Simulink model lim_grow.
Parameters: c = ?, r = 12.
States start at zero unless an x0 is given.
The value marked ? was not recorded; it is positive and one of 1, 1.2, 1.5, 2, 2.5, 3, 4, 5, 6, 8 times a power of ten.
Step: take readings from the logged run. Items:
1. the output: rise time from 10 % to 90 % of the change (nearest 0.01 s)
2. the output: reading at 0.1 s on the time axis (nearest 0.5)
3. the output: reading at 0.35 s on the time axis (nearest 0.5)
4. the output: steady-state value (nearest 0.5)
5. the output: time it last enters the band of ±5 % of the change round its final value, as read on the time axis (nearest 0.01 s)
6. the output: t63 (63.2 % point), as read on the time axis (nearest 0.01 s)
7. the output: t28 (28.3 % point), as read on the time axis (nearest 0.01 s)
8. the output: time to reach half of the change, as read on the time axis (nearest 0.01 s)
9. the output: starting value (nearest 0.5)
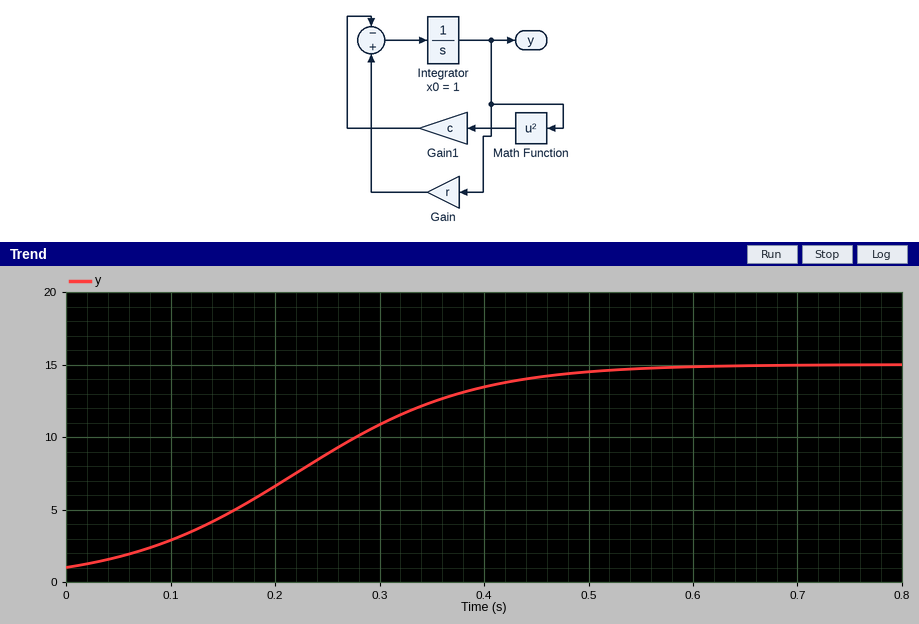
0.33 s
3.0
12.5
15.0
0.47 s
0.27 s
0.16 s
0.23 s
1.0
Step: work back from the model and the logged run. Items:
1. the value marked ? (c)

0.8
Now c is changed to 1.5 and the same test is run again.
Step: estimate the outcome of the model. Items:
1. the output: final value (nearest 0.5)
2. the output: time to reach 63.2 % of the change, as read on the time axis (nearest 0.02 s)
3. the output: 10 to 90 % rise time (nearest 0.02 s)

8.0
0.22 s
0.30 s
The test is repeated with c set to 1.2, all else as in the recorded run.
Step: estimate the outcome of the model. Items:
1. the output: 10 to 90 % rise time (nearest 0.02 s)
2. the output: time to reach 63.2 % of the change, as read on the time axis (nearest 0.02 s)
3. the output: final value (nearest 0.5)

0.32 s
0.24 s
10.0
